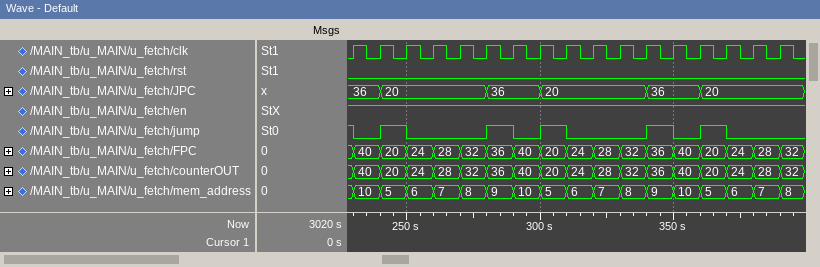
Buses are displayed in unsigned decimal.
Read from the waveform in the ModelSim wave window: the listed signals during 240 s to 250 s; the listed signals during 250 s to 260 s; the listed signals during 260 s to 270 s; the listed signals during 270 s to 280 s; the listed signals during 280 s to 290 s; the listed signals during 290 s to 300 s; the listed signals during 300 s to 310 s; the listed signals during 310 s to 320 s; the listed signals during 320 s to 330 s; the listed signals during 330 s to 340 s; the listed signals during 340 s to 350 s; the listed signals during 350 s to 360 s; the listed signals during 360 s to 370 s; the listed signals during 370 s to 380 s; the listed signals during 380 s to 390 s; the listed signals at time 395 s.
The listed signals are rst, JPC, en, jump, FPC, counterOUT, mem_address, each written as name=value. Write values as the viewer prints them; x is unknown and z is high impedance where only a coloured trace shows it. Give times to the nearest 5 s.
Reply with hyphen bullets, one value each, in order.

- rst=0, JPC=20, en=1, jump=1, FPC=20, counterOUT=20, mem_address=5
- rst=0, JPC=20, en=1, jump=0, FPC=24, counterOUT=24, mem_address=6
- rst=0, JPC=20, en=1, jump=0, FPC=28, counterOUT=28, mem_address=7
- rst=0, JPC=20, en=1, jump=0, FPC=32, counterOUT=32, mem_address=8
- rst=0, JPC=36, en=1, jump=1, FPC=36, counterOUT=36, mem_address=9
- rst=0, JPC=36, en=1, jump=0, FPC=40, counterOUT=40, mem_address=10
- rst=0, JPC=20, en=1, jump=1, FPC=20, counterOUT=20, mem_address=5
- rst=0, JPC=20, en=1, jump=0, FPC=24, counterOUT=24, mem_address=6
- rst=0, JPC=20, en=1, jump=0, FPC=28, counterOUT=28, mem_address=7
- rst=0, JPC=20, en=1, jump=0, FPC=32, counterOUT=32, mem_address=8
- rst=0, JPC=36, en=1, jump=1, FPC=36, counterOUT=36, mem_address=9
- rst=0, JPC=36, en=1, jump=0, FPC=40, counterOUT=40, mem_address=10
- rst=0, JPC=20, en=1, jump=1, FPC=20, counterOUT=20, mem_address=5
- rst=0, JPC=20, en=1, jump=0, FPC=24, counterOUT=24, mem_address=6
- rst=0, JPC=20, en=1, jump=0, FPC=28, counterOUT=28, mem_address=7
- rst=0, JPC=20, en=1, jump=0, FPC=32, counterOUT=32, mem_address=8
